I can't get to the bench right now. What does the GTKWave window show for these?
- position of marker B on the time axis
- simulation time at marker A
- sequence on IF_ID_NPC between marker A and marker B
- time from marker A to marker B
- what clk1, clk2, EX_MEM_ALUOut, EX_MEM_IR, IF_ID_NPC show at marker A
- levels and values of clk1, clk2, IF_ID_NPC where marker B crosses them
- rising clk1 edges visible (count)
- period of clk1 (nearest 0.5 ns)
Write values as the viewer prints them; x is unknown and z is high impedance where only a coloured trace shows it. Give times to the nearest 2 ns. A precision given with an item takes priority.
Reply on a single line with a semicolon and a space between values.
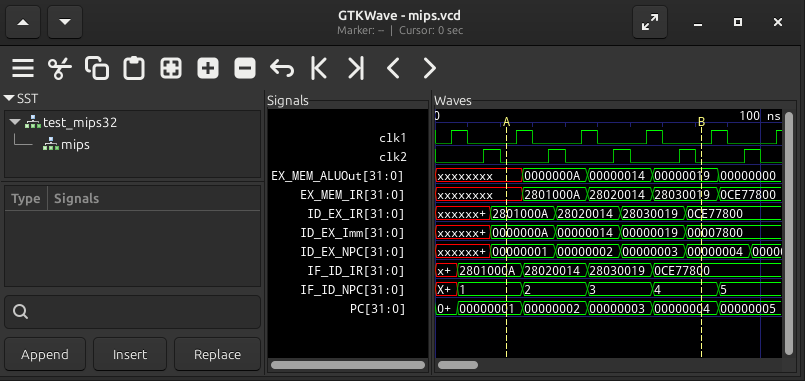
82 ns; 22 ns; 1, 2, 3, 4; 60 ns; clk1=0, clk2=0, EX_MEM_ALUOut=xxxxxxxx, EX_MEM_IR=xxxxxxxx, IF_ID_NPC=1; clk1=0, clk2=0, IF_ID_NPC=4; 6; 20 ns
